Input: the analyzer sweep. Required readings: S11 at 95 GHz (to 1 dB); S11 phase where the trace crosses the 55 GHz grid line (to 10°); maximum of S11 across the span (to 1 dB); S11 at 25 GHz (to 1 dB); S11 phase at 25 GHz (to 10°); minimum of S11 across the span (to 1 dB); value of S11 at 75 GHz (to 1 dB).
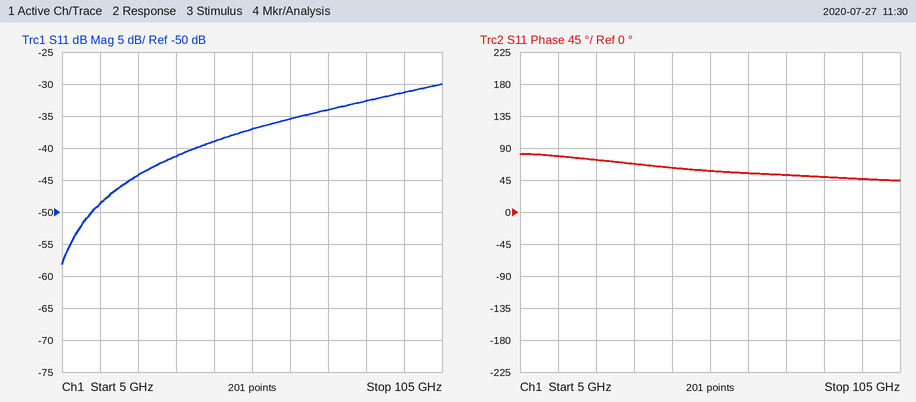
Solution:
-31 dB
60°
-30 dB
-44 dB
70°
-58 dB
-34 dB
